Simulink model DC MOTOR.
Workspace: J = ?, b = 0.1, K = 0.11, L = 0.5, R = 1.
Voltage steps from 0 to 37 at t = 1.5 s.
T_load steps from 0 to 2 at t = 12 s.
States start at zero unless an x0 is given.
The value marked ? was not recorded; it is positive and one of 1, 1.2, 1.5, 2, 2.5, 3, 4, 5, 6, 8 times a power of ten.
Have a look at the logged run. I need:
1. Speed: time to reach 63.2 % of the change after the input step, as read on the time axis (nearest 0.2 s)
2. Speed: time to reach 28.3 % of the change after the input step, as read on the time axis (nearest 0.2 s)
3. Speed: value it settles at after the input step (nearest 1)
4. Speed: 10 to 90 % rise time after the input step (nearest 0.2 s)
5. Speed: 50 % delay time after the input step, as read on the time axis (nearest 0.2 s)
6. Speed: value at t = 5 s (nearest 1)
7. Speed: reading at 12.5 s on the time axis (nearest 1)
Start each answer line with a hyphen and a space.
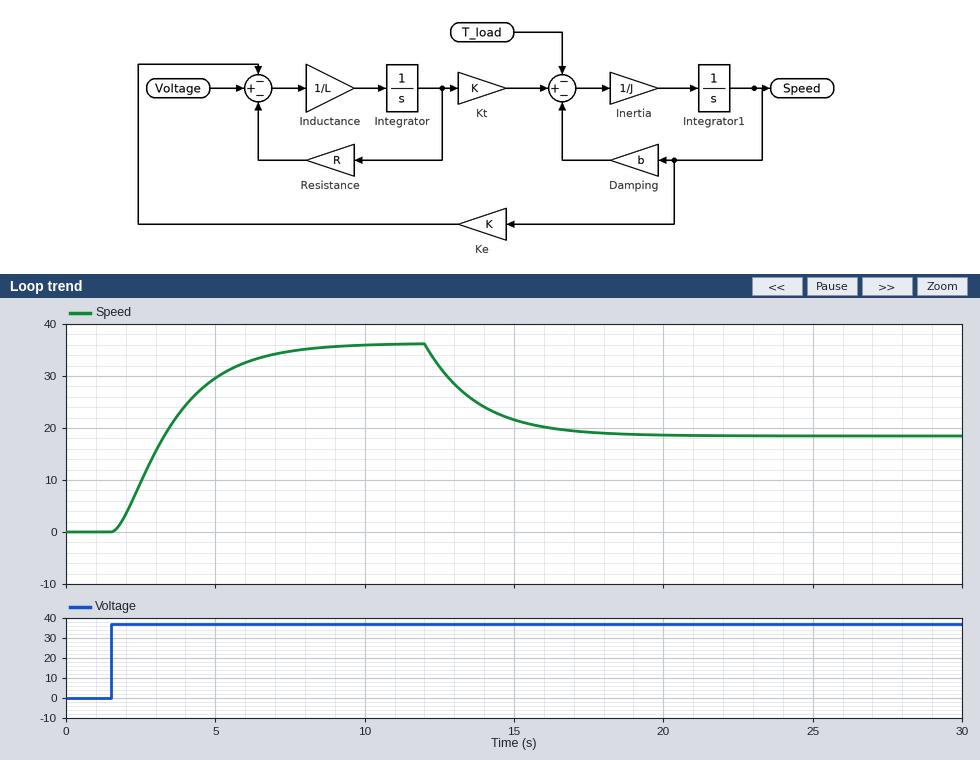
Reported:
- 3.8 s
- 2.6 s
- 36
- 4.0 s
- 3.2 s
- 30
- 32
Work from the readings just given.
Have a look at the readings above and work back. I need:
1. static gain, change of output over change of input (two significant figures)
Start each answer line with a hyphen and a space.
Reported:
- 0.97
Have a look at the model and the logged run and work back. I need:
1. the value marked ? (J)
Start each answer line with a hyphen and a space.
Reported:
- 0.2
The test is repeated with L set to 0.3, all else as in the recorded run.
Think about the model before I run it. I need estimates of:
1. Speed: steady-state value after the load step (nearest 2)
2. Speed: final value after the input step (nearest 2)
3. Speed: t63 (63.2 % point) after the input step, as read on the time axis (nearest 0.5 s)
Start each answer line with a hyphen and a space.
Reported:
- 18
- 36
- 3.5 s
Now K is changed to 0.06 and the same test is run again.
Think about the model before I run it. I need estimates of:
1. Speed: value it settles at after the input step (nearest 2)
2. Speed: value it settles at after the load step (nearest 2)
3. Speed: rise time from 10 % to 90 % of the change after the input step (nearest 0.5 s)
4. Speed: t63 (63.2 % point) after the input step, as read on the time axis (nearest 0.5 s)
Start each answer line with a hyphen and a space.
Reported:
- 22
- 2
- 4.5 s
- 4.0 s
